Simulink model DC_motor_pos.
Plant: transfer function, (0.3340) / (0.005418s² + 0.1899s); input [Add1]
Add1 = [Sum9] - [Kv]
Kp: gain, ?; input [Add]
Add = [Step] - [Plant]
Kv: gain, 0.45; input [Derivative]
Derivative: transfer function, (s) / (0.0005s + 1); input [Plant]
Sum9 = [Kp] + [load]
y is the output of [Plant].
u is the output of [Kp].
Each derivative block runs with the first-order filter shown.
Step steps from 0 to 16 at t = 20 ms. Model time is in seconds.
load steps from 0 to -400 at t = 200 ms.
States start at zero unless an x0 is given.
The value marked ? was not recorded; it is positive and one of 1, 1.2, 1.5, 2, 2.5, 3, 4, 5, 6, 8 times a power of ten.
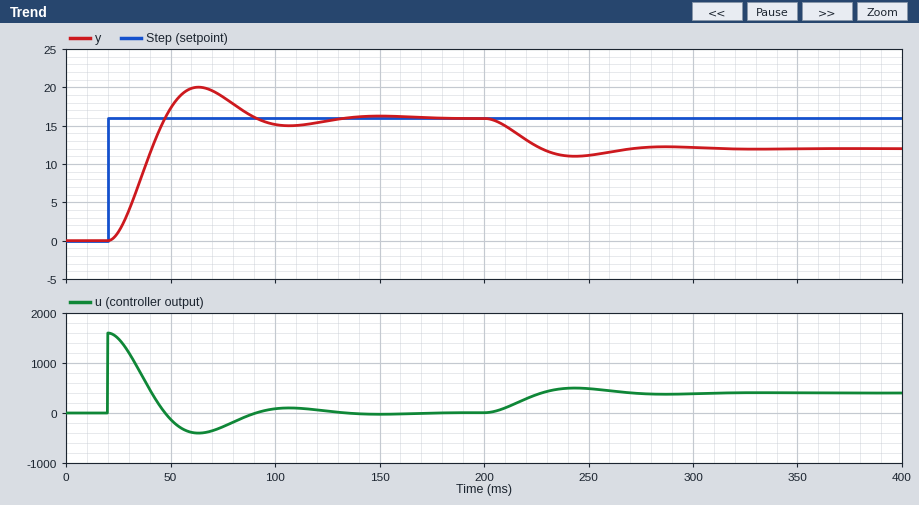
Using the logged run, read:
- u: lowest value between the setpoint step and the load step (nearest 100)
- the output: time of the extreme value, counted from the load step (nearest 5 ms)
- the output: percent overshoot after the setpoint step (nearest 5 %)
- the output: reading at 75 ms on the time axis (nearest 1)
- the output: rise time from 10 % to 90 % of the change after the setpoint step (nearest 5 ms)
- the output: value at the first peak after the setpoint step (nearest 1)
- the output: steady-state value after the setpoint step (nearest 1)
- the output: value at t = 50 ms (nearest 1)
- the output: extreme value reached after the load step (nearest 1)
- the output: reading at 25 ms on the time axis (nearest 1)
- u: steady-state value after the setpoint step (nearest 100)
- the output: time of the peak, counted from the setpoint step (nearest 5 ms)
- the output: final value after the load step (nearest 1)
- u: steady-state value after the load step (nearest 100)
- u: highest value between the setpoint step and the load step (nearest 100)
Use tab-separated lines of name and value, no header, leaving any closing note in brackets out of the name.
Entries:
u: lowest value between the setpoint step and the load step	-400
the output: time of the extreme value, counted from the load step	45 ms
the output: percent overshoot after the setpoint step	25 %
the output: reading at 75 ms on the time axis	19
the output: rise time from 10 % to 90 % of the change after the setpoint step	20 ms
the output: value at the first peak after the setpoint step	20
the output: steady-state value after the setpoint step	16
the output: value at t = 50 ms	17
the output: extreme value reached after the load step	11
the output: reading at 25 ms on the time axis	1
u: steady-state value after the setpoint step	0
the output: time of the peak, counted from the setpoint step	45 ms
the output: final value after the load step	12
u: steady-state value after the load step	400
u: highest value between the setpoint step and the load step	1600
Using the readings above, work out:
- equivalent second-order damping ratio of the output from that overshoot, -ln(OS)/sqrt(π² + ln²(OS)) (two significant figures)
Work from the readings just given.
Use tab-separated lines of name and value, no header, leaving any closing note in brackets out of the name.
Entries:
equivalent second-order damping ratio of the output from that overshoot, -ln(OS)/sqrt(π² + ln²(OS))	0.40
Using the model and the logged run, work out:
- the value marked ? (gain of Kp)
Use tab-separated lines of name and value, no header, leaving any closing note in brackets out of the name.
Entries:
the value marked ?	100
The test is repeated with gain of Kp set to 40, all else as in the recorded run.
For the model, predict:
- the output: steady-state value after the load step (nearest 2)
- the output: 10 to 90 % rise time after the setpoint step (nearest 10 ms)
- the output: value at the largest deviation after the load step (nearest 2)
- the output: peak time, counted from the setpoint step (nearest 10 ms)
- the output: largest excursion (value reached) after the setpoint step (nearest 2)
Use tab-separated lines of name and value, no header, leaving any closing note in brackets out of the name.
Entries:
the output: steady-state value after the load step	6
the output: 10 to 90 % rise time after the setpoint step	40 ms
the output: value at the largest deviation after the load step	6
the output: peak time, counted from the setpoint step	80 ms
the output: largest excursion (value reached) after the setpoint step	18
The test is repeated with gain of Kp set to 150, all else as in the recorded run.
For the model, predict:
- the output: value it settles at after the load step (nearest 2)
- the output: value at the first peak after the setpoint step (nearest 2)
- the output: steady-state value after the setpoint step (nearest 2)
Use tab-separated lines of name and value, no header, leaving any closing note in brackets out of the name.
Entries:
the output: value it settles at after the load step	14
the output: value at the first peak after the setpoint step	22
the output: steady-state value after the setpoint step	16
